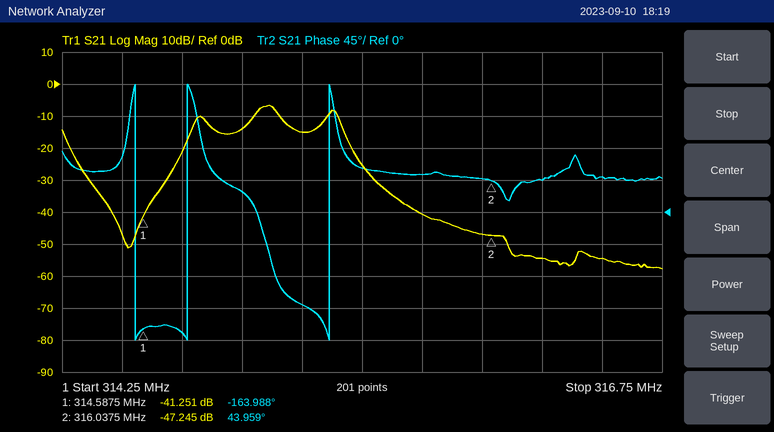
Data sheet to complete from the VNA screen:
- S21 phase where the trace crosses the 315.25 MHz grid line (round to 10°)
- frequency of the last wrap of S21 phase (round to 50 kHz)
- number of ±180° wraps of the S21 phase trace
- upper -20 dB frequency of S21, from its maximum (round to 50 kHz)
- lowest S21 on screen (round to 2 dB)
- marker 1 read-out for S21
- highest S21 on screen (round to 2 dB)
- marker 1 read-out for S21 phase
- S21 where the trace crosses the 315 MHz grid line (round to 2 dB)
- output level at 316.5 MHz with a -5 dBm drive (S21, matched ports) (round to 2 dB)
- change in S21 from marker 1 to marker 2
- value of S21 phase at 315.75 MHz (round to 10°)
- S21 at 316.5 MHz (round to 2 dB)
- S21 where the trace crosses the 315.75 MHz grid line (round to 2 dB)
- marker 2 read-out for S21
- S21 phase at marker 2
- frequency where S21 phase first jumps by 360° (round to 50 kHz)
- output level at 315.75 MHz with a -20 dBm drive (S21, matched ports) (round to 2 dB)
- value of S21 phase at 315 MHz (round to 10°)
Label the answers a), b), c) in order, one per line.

a) -130°
b) 315.35 MHz
c) 3
d) 315.50 MHz
e) -58 dB
f) -41.251 dB
g) -6 dB
h) -163.988°
i) -14 dB
j) -60 dBm
k) -5.994 dB
l) 50°
m) -54 dB
n) -40 dB
o) -47.245 dB
p) 43.959°
q) 314.55 MHz
r) -60 dBm
s) 30°
